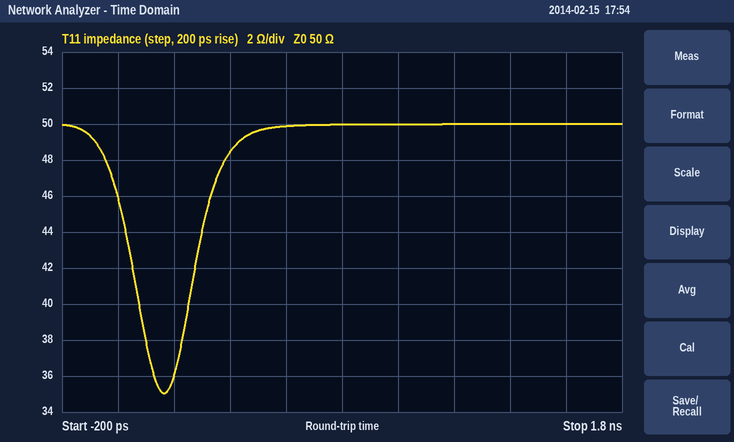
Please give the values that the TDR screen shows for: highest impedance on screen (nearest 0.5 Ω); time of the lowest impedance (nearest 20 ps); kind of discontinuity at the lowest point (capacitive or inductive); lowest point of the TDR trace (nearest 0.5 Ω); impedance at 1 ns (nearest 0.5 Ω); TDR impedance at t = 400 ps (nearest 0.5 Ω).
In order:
50.0 Ω
160 ps
capacitive
35.0 Ω
50.0 Ω
48.5 Ω
